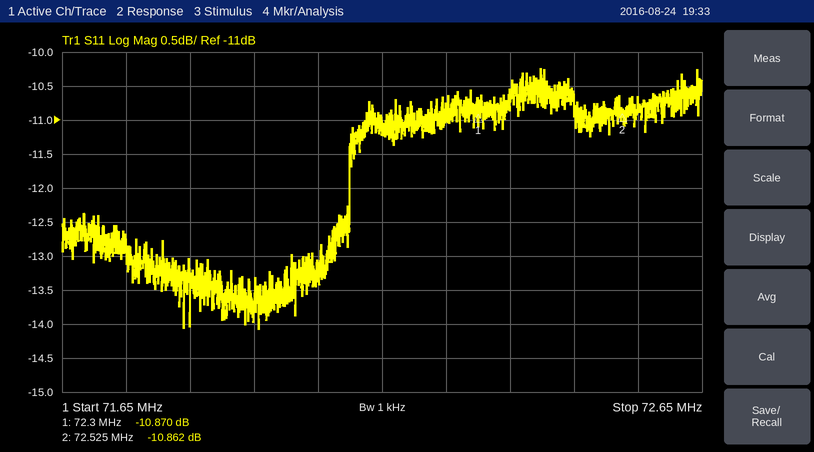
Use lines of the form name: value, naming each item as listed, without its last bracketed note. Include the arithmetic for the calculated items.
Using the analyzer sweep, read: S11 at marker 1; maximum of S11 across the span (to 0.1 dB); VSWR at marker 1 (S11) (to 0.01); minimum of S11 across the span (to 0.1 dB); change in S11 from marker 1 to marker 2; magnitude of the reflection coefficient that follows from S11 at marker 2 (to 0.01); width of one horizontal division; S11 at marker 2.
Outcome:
S11 at marker 1: -10.870 dB
maximum of S11 across the span: -10.2 dB
VSWR at marker 1 (S11): (1 + 0.2861)/(1 − 0.2861) ≈ 1.80
minimum of S11 across the span: -14.1 dB
change in S11 from marker 1 to marker 2: -10.862 − (-10.87) = 0.008 dB
magnitude of the reflection coefficient that follows from S11 at marker 2: 10^(-10.862/20) ≈ 0.29
width of one horizontal division: 100 kHz
S11 at marker 2: -10.862 dB
